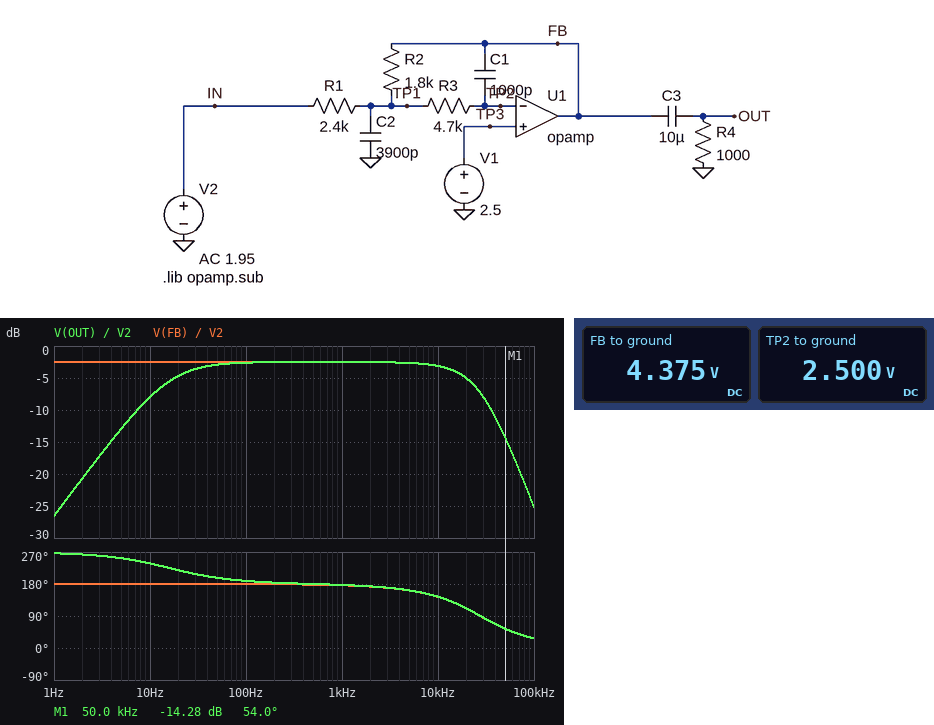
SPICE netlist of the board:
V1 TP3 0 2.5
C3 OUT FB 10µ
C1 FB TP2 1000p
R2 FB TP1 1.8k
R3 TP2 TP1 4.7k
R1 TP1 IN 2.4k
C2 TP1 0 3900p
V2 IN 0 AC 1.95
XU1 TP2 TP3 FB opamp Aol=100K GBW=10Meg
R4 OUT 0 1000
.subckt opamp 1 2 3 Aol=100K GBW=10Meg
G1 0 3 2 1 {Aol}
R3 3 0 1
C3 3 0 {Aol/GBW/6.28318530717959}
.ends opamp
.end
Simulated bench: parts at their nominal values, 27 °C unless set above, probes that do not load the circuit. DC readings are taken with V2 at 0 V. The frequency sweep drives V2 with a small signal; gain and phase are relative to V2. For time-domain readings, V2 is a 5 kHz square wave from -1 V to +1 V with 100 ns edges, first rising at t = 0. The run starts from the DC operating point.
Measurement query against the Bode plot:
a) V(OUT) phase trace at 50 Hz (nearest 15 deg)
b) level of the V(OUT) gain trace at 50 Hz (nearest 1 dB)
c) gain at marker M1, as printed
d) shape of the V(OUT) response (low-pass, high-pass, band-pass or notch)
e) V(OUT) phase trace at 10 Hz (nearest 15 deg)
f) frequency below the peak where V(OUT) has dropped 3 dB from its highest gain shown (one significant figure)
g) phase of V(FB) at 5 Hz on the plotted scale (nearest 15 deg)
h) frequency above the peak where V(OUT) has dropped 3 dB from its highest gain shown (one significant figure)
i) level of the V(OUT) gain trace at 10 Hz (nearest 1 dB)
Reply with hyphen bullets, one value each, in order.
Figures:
- 195 deg
- -3 dB
- -14.28 dB
- band-pass
- 240 deg
- 20 Hz
- 180 deg
- 20 kHz
- -8 dB
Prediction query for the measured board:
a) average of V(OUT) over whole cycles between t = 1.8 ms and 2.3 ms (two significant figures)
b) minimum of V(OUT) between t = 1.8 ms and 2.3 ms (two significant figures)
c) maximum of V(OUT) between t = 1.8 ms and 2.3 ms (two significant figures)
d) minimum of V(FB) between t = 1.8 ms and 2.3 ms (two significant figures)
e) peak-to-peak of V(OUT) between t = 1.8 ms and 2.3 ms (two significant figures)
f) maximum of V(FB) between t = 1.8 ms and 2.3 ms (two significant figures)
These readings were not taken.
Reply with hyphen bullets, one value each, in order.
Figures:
- -610 mV
- -1.4 V
- 150 mV
- 3.6 V
- 1.5 V
- 5.1 V
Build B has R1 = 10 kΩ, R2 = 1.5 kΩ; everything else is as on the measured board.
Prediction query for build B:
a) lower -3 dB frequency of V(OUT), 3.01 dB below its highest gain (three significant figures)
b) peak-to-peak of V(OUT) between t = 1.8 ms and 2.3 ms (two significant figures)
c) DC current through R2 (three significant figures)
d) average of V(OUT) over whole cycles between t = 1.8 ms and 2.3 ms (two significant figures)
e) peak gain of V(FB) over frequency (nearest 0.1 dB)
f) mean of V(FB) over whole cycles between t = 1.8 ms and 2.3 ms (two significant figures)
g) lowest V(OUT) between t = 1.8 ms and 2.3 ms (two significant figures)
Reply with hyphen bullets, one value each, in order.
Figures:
- 16.2 Hz
- 340 mV
- 250 µA
- -120 mV
- -16.4 dB
- 2.9 V
- -290 mV
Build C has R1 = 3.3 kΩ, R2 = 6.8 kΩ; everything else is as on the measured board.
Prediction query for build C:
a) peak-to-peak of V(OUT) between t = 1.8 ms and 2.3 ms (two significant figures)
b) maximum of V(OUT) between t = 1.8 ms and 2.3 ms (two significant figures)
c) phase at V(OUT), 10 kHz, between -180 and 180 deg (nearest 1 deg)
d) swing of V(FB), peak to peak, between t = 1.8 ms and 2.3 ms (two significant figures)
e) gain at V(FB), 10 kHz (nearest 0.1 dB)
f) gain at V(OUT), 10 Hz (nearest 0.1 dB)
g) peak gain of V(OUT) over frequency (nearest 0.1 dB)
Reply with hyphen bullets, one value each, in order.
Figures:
- 4.2 V
- 410 mV
- 111 deg
- 4.1 V
- 3.2 dB
- 0.8 dB
- 6.3 dB
